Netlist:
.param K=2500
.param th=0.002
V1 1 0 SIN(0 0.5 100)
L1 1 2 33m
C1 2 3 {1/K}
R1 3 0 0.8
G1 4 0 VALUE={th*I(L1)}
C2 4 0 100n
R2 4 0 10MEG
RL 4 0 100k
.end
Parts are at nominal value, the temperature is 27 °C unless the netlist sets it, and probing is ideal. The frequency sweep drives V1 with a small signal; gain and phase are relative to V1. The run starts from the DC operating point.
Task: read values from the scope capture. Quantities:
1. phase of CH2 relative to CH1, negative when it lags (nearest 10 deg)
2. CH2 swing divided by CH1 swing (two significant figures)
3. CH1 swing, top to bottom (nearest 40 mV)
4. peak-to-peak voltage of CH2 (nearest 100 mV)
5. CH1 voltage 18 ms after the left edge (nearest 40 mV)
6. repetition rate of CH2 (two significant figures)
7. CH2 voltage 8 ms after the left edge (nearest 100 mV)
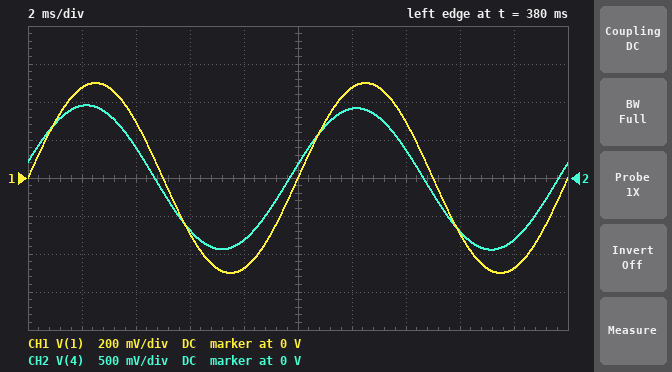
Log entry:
10 deg
1.9
1.00 V
1.9 V
-480 mV
100 Hz
-800 mV
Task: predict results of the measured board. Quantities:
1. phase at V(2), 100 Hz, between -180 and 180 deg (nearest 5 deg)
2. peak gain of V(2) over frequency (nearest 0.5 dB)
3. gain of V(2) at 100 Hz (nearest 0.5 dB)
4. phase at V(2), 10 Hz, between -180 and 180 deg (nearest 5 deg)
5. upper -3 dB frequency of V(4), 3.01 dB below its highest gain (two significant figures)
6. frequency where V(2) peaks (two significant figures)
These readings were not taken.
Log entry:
-165 deg
21.0 dB
-12.5 dB
0 deg
46 Hz
44 Hz
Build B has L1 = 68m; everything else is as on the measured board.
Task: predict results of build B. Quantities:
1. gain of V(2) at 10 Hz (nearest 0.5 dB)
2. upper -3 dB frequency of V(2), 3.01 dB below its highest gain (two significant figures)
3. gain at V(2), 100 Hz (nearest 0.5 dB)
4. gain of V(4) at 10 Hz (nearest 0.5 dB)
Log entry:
1.0 dB
31 Hz
-19.5 dB
13.5 dB
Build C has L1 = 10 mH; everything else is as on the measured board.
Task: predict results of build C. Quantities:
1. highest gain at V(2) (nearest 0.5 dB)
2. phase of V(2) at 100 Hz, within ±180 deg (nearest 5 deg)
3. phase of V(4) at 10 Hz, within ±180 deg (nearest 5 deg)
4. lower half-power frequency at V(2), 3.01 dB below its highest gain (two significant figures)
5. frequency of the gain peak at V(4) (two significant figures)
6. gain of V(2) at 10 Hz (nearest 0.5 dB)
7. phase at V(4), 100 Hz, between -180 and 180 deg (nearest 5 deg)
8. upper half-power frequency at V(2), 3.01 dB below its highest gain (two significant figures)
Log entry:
16.0 dB
-150 deg
-125 deg
72 Hz
79 Hz
0 dB
30 deg
85 Hz
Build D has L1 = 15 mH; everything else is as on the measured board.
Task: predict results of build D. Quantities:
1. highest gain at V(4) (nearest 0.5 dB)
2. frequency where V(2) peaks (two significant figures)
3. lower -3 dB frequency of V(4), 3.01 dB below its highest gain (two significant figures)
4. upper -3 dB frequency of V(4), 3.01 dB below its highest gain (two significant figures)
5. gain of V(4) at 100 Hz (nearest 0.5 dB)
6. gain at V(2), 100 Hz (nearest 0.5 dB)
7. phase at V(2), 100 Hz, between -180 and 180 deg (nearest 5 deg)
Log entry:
35.5 dB
65 Hz
60 Hz
69 Hz
15.0 dB
-2.5 dB
-160 deg
